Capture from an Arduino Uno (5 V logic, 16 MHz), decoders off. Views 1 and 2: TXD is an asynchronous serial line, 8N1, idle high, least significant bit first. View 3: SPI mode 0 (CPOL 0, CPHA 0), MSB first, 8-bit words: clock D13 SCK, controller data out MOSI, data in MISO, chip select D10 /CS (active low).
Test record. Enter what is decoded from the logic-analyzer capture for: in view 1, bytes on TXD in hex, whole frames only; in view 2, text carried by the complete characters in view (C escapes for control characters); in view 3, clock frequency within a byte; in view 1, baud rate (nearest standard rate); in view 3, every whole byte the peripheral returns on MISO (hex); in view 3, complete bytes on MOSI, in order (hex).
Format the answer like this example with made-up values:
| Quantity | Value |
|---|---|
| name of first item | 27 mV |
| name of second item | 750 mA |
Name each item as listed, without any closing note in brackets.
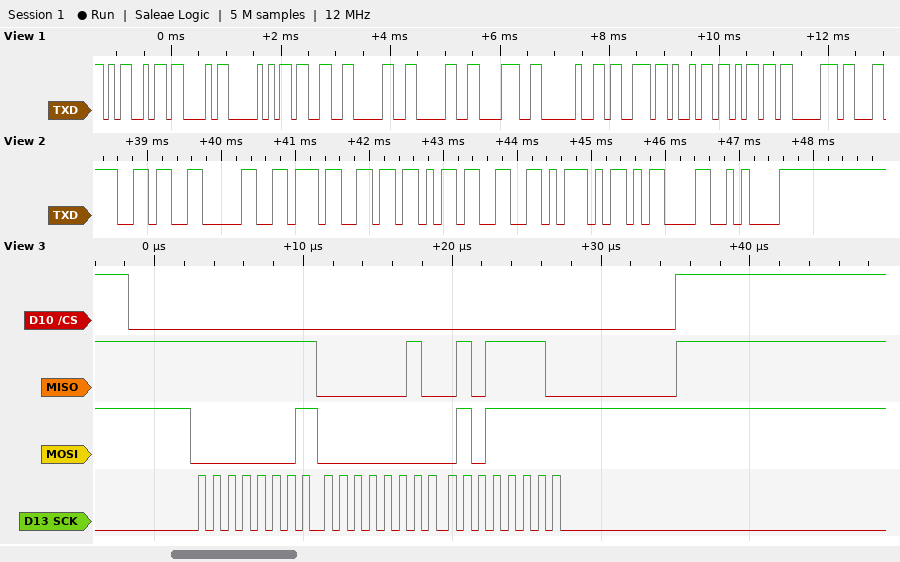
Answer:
| Quantity | Value |
|---|---|
| in view 1, bytes on TXD in hex, whole frames only | 0x4D 0x43 0x50 0x33 0x30 0x30 0x38 0x20 0x73 0x69 0x6D 0x70 |
| in view 2, text carried by the complete characters in view | "607[3]\r\n" |
| in view 3, clock frequency within a byte | 1 MHz |
| in view 1, baud rate | 9600 baud |
| in view 3, every whole byte the peripheral returns on MISO | FF 02 5E |
| in view 3, complete bytes on MOSI, in order | 01 00 5F |
